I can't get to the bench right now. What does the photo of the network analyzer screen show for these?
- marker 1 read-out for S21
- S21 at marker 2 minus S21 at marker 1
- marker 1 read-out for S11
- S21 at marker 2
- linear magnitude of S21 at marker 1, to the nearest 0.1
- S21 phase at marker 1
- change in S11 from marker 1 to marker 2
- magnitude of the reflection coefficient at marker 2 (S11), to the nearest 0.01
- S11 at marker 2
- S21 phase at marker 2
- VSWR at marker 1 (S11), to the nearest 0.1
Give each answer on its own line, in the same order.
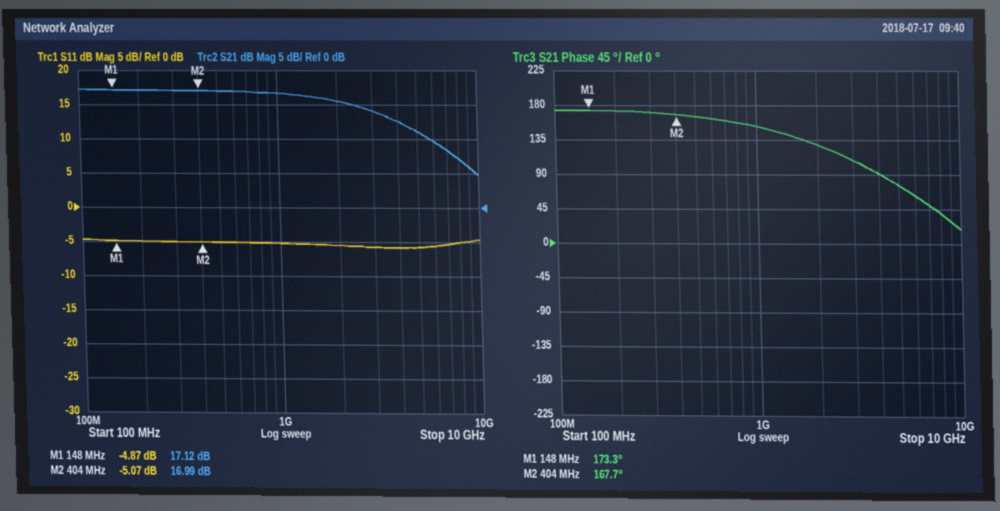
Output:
17.12 dB
-0.13 dB
-4.87 dB
16.99 dB
7.2
173.3°
-0.20 dB
0.56
-5.07 dB
167.7°
3.7
